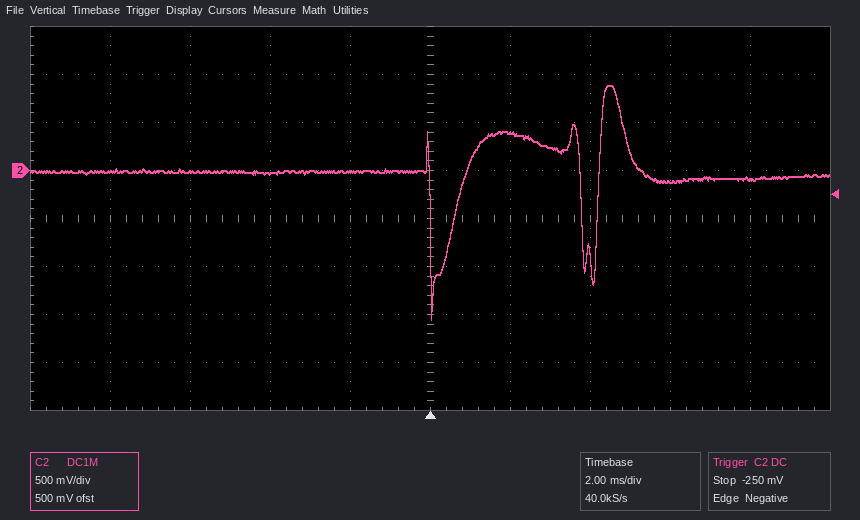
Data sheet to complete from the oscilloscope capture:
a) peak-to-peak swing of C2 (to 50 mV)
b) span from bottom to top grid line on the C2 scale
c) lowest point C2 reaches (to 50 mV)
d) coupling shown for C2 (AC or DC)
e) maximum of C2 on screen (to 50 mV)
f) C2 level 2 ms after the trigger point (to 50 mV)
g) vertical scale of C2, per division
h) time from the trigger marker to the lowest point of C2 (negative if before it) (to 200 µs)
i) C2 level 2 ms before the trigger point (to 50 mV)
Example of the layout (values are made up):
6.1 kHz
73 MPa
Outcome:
2.45 V
4 V
-1.55 V
DC
900 mV
400 mV
500 mV
0.0 ms
0 mV
